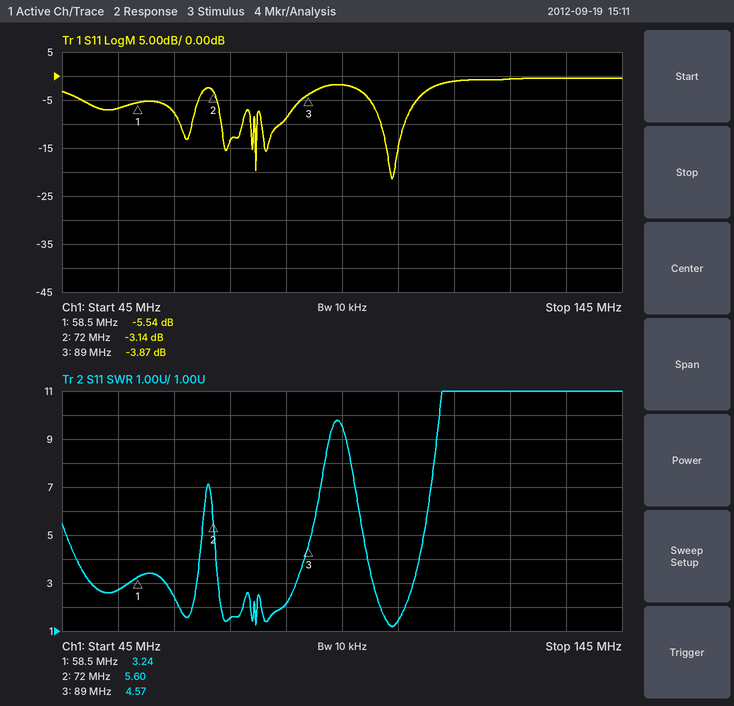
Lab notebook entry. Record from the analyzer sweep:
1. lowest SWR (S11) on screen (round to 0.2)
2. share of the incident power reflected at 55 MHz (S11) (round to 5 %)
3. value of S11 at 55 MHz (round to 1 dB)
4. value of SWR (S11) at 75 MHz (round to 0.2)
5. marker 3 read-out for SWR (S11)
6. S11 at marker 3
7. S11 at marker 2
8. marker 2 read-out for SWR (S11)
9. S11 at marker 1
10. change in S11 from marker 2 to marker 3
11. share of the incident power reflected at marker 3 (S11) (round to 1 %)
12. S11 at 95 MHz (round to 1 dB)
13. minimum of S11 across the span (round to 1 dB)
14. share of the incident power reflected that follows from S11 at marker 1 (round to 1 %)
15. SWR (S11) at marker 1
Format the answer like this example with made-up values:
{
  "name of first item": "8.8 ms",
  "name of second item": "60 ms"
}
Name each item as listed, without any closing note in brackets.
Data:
{
  "lowest SWR (S11) on screen": "1.2",
  "share of the incident power reflected at 55 MHz (S11)": "20 %",
  "value of S11 at 55 MHz": "-7 dB",
  "value of SWR (S11) at 75 MHz": "1.6",
  "marker 3 read-out for SWR": "4.57",
  "S11 at marker 3": "-3.87 dB",
  "S11 at marker 2": "-3.14 dB",
  "marker 2 read-out for SWR": "5.60",
  "S11 at marker 1": "-5.54 dB",
  "change in S11 from marker 2 to marker 3": "-0.73 dB",
  "share of the incident power reflected at marker 3 (S11)": "41 %",
  "S11 at 95 MHz": "-2 dB",
  "minimum of S11 across the span": "-21 dB",
  "share of the incident power reflected that follows from S11 at marker 1": "28 %",
  "SWR (S11) at marker 1": "3.24"
}
